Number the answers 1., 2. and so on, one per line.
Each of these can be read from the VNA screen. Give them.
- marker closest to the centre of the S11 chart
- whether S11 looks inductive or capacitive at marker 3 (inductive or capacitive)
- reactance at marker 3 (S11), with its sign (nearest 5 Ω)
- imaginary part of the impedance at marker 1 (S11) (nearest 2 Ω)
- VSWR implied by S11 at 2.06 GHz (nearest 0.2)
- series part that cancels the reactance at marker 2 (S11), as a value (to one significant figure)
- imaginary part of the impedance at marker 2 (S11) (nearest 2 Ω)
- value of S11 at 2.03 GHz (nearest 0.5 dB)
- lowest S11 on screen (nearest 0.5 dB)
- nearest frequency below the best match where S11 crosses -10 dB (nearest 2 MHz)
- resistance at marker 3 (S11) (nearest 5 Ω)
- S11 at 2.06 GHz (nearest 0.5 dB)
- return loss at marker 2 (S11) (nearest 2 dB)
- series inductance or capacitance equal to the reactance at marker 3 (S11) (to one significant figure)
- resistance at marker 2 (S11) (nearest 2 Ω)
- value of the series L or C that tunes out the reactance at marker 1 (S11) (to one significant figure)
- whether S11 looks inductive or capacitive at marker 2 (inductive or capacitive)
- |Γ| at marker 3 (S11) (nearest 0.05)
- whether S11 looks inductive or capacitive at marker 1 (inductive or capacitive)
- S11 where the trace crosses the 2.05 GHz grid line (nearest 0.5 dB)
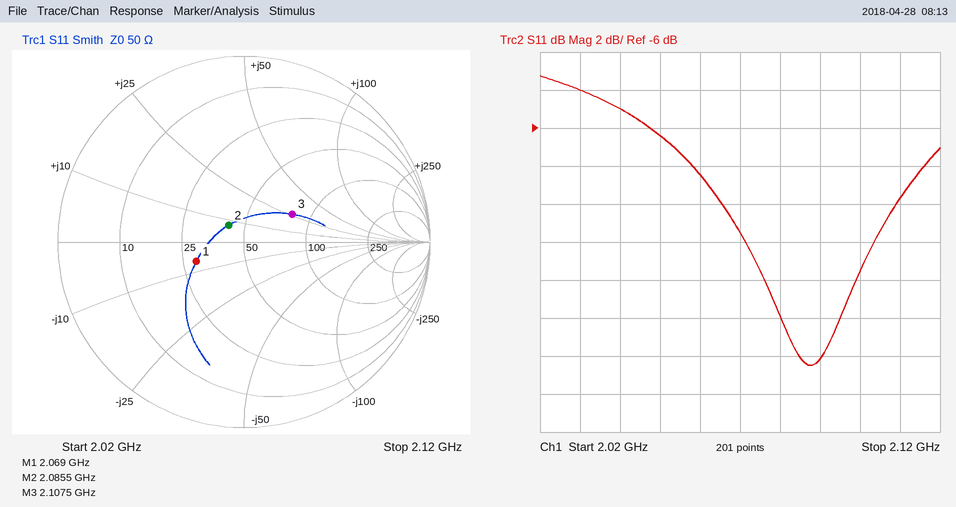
1. marker 2
2. inductive
3. +25 Ω
4. -6 Ω
5. 2.2
6. 10 pF
7. +8 Ω
8. -4.0 dB
9. -18.5 dB
10. 2.066 GHz
11. 80 Ω
12. -8.5 dB
13. 18 dB
14. 2 nH
15. 42 Ω
16. 500 pH
17. inductive
18. 0.30
19. capacitive
20. -6.5 dB
